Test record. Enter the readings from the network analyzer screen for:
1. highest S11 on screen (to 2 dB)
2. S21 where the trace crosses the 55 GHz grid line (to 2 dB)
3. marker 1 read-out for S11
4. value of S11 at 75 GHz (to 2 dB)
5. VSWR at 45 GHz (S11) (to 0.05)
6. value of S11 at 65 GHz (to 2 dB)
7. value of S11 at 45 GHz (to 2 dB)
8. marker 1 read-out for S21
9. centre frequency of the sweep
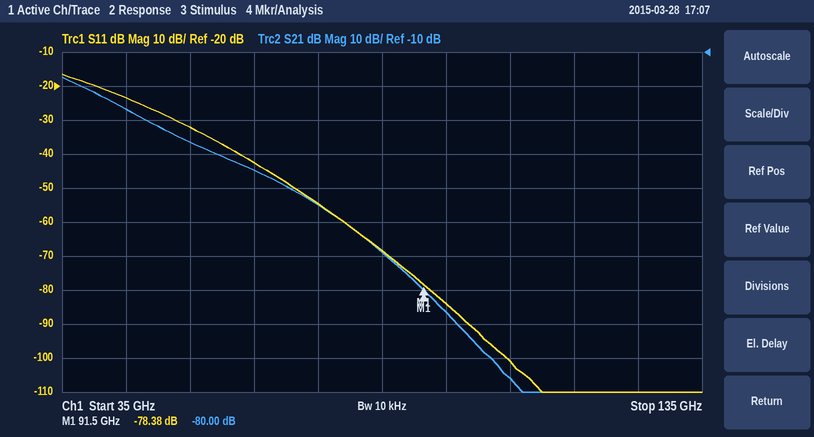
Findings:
-16 dB
-36 dB
-78.38 dB
-54 dB
1.15
-42 dB
-24 dB
-80.00 dB
85 GHz
